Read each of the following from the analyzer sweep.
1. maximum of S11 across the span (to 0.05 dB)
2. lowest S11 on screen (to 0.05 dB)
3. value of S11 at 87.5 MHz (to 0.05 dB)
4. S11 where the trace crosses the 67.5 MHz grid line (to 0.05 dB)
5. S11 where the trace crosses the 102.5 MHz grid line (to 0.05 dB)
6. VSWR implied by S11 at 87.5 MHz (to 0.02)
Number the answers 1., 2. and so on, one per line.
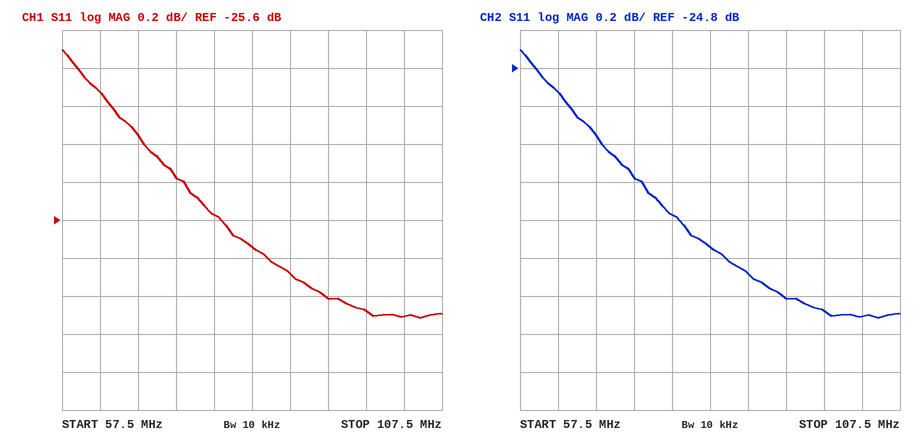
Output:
1. -24.70 dB
2. -26.10 dB
3. -25.90 dB
4. -25.15 dB
5. -26.10 dB
6. 1.10
